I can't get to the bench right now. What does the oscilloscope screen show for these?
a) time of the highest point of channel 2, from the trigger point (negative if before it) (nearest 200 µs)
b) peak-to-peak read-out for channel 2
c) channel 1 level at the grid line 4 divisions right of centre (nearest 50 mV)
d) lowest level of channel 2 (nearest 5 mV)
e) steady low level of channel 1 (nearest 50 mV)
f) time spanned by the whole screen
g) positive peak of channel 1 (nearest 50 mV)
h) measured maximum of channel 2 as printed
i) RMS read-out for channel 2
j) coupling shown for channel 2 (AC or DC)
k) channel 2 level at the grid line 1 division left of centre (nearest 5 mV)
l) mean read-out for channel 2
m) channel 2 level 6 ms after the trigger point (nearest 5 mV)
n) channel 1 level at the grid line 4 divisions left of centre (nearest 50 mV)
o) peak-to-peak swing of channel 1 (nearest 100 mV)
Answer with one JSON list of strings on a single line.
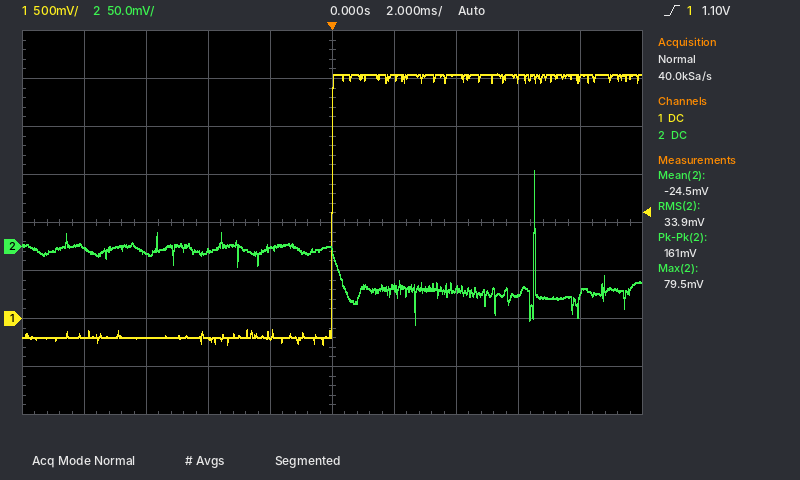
["+6.6 ms", "161 mV", "2.50 V", "-80 mV", "-200 mV", "20 ms", "2.55 V", "79.5 mV", "33.9 mV", "DC", "0 mV", "-24.5 mV", "-50 mV", "-200 mV", "2.80 V"]
